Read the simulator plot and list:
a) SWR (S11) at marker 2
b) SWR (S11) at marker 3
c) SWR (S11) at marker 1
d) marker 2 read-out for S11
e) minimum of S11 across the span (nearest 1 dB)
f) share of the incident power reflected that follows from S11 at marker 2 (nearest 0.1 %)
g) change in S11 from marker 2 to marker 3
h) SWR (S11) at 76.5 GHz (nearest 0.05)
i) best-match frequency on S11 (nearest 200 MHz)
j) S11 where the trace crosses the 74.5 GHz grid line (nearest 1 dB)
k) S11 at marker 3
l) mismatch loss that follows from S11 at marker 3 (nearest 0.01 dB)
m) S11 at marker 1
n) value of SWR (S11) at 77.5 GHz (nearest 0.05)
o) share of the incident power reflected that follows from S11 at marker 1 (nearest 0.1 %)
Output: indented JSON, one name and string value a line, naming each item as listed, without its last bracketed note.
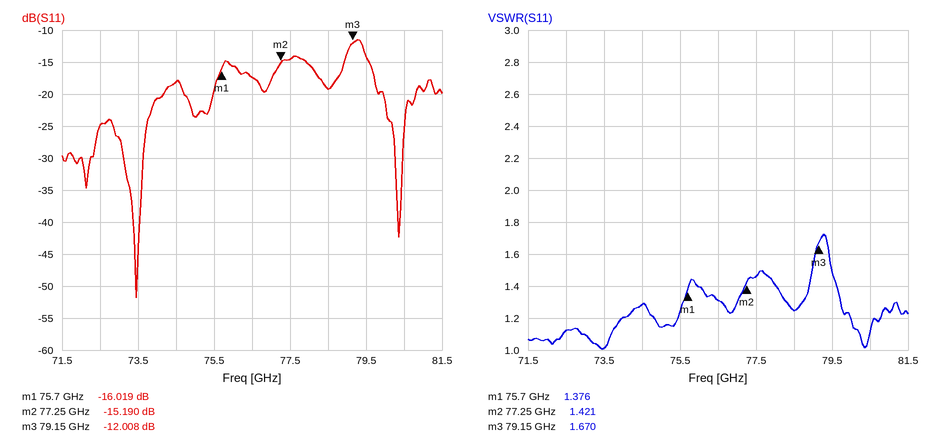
{
  "SWR (S11) at marker 2": "1.421",
  "SWR (S11) at marker 3": "1.670",
  "SWR (S11) at marker 1": "1.376",
  "marker 2 read-out for S11": "-15.190 dB",
  "minimum of S11 across the span": "-52 dB",
  "share of the incident power reflected that follows from S11 at marker 2": "3.0 %",
  "change in S11 from marker 2 to marker 3": "3.182 dB",
  "SWR (S11) at 76.5 GHz": "1.30",
  "best-match frequency on S11": "73.4 GHz",
  "S11 where the trace crosses the 74.5 GHz grid line": "-18 dB",
  "S11 at marker 3": "-12.008 dB",
  "mismatch loss that follows from S11 at marker 3": "0.28 dB",
  "S11 at marker 1": "-16.019 dB",
  "value of SWR (S11) at 77.5 GHz": "1.45",
  "share of the incident power reflected that follows from S11 at marker 1": "2.5 %"
}
